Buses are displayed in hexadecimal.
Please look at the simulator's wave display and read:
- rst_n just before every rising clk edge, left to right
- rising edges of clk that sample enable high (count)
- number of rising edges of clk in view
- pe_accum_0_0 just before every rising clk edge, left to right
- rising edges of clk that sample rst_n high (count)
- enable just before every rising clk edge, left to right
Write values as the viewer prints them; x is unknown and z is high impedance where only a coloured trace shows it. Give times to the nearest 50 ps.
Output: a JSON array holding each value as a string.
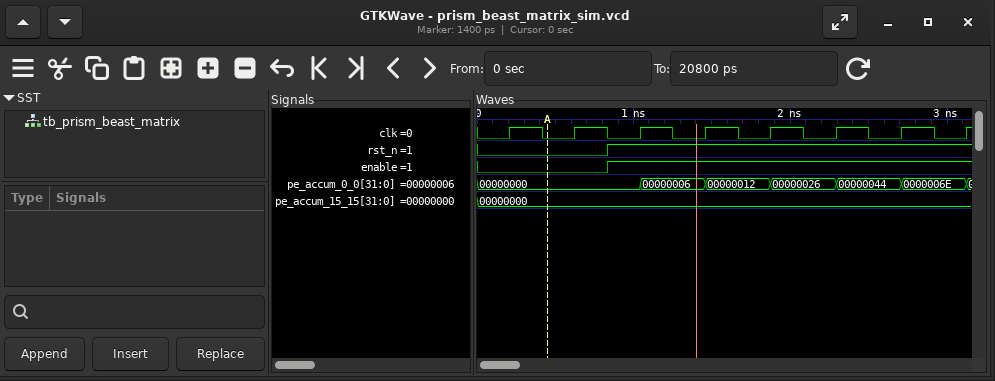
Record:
["0 0 1 1 1 1 1 1", "6", "8", "00000000, 00000000, 00000000, 00000006, 00000012, 00000026, 00000044, 0000006E", "6", "0 0 1 1 1 1 1 1"]
